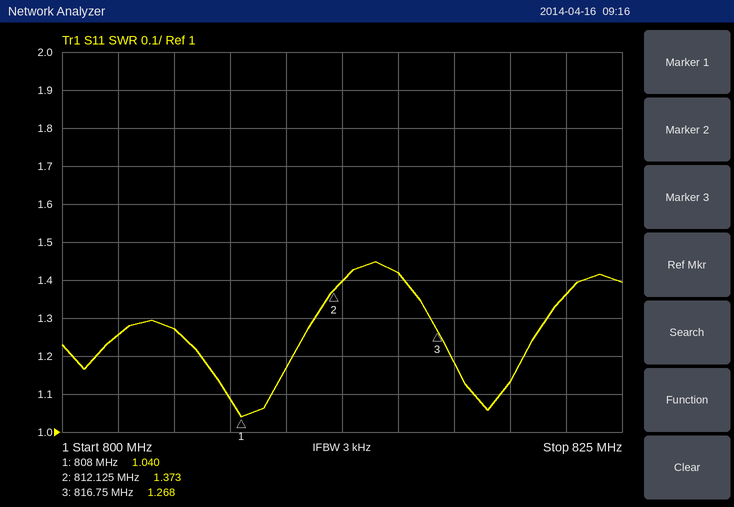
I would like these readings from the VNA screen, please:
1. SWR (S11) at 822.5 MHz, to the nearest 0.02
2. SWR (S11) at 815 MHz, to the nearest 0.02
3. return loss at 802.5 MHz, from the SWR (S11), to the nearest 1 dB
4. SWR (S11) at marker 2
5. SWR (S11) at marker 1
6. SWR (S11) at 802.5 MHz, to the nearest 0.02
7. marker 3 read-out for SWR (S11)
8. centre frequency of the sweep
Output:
1.36
1.42
19 dB
1.373
1.040
1.26
1.268
812.5 MHz
